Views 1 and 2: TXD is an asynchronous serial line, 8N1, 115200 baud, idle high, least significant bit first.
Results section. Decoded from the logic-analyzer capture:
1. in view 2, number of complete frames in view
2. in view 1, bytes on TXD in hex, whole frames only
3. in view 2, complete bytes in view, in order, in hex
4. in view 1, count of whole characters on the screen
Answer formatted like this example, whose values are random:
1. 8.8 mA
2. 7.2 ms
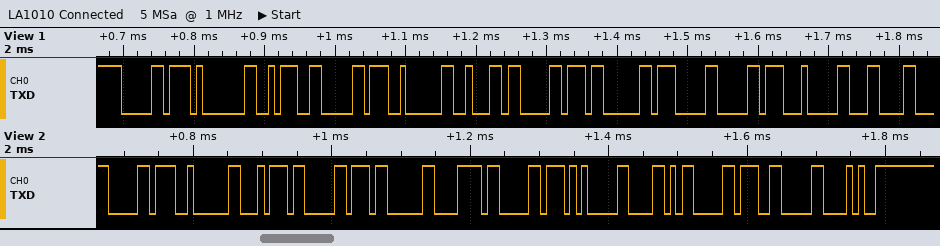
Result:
1. 12
2. B0 01 3A B0 02 62 B0 03 07 B0 04 0C
3. 0xB0 0x02 0x74 0xB0 0x03 0x78 0xB0 0x05 0x58 0xB0 0x06 0x28
4. 12
